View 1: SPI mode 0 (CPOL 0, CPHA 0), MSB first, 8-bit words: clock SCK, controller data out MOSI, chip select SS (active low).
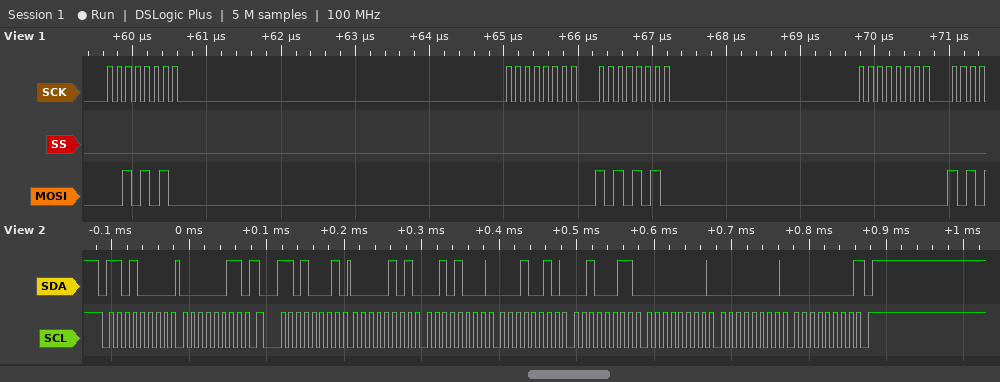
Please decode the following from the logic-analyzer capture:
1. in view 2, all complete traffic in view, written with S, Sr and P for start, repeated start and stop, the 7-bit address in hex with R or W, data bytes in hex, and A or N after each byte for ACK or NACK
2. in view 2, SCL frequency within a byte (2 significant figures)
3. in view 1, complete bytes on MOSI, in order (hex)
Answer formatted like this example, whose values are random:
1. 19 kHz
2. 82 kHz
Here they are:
1. S 68W A 03 A Sr 68R A 05 A 28 A 12 A 23 A 00 A 00 A 00 N P
2. 100 kHz
3. 2A 00 AA 00
